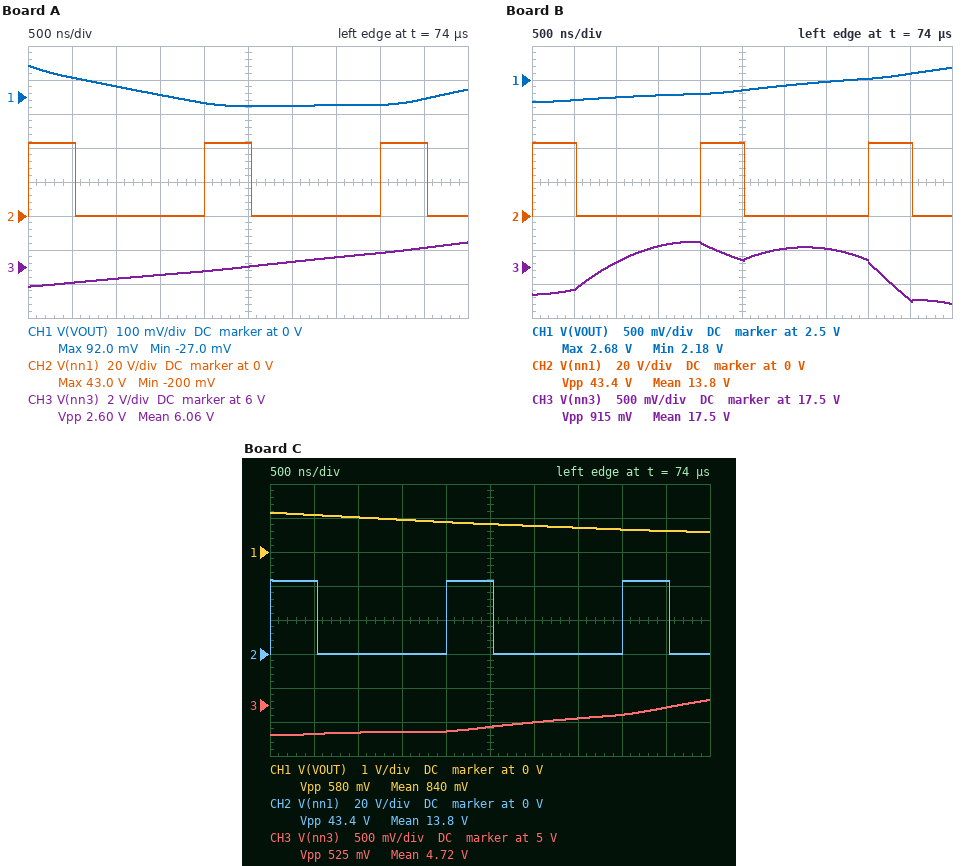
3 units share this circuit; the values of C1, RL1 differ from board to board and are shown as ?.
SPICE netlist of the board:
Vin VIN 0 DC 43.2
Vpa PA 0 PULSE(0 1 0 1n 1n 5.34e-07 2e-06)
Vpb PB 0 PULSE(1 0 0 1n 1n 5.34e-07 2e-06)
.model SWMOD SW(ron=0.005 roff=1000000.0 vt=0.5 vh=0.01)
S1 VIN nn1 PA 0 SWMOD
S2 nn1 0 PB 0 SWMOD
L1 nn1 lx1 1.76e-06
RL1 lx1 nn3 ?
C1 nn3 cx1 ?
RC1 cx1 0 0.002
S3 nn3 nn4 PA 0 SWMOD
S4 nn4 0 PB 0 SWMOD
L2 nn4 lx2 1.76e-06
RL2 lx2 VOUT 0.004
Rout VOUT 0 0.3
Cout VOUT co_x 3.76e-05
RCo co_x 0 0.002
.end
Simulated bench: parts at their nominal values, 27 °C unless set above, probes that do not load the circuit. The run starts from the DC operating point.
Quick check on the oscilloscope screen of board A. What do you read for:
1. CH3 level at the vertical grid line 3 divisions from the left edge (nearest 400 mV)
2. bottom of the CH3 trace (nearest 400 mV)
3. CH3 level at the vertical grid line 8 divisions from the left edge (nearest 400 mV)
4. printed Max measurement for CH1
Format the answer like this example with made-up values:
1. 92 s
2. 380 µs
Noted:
1. 5.6 V
2. 4.8 V
3. 6.8 V
4. 92.0 mV
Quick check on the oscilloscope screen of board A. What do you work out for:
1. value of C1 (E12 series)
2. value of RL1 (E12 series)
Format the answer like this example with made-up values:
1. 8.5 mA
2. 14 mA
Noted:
1. 68 µF
2. 1.2 mΩ
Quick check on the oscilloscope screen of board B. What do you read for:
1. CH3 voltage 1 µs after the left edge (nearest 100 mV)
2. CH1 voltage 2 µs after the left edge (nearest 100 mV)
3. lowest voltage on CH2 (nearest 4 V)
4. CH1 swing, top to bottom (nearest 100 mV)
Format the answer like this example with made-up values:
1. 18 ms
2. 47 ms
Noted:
1. 17.6 V
2. 2.3 V
3. 0 V
4. 500 mV
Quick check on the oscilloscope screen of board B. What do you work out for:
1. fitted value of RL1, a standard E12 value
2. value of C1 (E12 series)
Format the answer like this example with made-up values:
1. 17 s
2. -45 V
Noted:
1. 0.01 Ω
2. 15 µF
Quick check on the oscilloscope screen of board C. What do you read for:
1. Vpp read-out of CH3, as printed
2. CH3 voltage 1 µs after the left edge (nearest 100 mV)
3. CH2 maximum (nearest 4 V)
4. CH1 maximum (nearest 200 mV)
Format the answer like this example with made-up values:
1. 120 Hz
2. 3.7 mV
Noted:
1. 525 mV
2. 4.6 V
3. 44 V
4. 1.2 V
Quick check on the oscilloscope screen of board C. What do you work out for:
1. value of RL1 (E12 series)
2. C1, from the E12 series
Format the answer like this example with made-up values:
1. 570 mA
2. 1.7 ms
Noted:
1. 8.2 mΩ
2. 82 µF
